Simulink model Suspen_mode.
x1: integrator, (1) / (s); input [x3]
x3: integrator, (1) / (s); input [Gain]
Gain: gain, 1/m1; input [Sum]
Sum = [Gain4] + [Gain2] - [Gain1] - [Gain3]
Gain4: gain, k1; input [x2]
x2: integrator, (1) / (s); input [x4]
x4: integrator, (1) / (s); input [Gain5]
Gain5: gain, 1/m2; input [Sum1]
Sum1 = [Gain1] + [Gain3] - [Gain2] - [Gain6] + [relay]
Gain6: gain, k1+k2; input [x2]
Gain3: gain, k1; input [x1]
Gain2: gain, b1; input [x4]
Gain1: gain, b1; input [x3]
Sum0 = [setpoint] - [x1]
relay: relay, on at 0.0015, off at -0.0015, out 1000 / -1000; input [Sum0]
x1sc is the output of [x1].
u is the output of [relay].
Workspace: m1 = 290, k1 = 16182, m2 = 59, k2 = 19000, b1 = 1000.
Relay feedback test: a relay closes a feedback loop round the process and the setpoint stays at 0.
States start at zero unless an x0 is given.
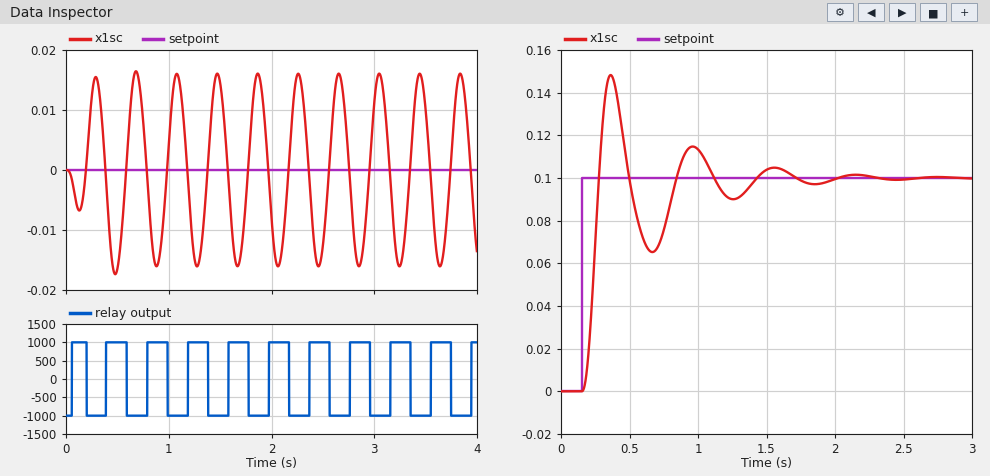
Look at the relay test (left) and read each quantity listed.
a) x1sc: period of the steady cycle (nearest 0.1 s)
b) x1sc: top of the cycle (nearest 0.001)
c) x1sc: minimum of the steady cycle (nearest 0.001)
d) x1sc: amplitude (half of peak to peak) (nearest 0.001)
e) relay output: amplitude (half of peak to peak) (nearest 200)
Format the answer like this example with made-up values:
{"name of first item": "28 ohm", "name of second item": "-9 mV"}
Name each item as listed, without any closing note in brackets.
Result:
{"x1sc: period of the steady cycle": "0.4 s", "x1sc: top of the cycle": "0.016", "x1sc: minimum of the steady cycle": "-0.016", "x1sc: amplitude (half of peak to peak)": "0.016", "relay output: amplitude (half of peak to peak)": "1000"}
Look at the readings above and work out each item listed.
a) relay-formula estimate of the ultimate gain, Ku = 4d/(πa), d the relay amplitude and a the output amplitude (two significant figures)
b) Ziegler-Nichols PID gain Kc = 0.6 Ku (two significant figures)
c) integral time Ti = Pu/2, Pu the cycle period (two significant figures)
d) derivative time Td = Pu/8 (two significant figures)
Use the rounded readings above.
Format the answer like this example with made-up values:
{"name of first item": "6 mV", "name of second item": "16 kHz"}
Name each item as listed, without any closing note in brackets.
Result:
{"relay-formula estimate of the ultimate gain, Ku = 4d/(πa), d the relay amplitude and a the output amplitude": "80000", "Ziegler-Nichols PID gain Kc = 0.6 Ku": "48000", "integral time Ti = Pu/2, Pu the cycle period": "0.20 s", "derivative time Td = Pu/8": "0.050 s"}
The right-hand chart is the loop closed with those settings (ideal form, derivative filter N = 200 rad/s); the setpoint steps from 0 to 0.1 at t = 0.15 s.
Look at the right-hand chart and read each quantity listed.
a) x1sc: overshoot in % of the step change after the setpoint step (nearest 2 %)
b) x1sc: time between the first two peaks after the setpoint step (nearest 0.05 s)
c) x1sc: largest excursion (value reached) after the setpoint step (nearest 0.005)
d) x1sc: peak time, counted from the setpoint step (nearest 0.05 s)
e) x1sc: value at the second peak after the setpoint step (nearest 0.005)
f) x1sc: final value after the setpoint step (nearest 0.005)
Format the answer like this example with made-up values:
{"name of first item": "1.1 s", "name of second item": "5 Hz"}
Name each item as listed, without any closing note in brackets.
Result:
{"x1sc: overshoot in % of the step change after the setpoint step": "48 %", "x1sc: time between the first two peaks after the setpoint step": "0.60 s", "x1sc: largest excursion (value reached) after the setpoint step": "0.150", "x1sc: peak time, counted from the setpoint step": "0.20 s", "x1sc: value at the second peak after the setpoint step": "0.115", "x1sc: final value after the setpoint step": "0.100"}
